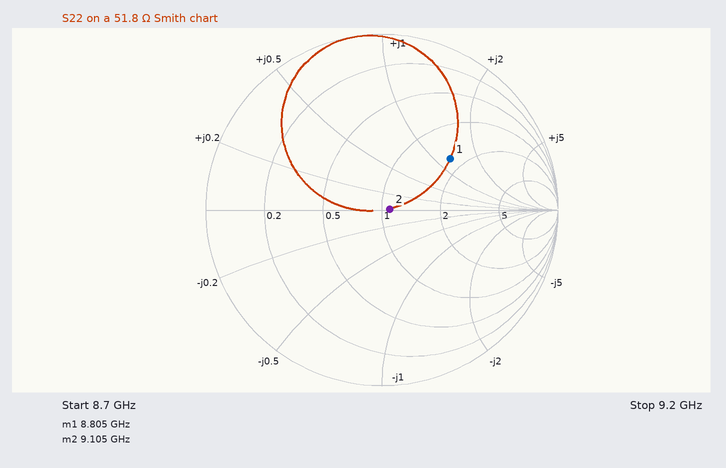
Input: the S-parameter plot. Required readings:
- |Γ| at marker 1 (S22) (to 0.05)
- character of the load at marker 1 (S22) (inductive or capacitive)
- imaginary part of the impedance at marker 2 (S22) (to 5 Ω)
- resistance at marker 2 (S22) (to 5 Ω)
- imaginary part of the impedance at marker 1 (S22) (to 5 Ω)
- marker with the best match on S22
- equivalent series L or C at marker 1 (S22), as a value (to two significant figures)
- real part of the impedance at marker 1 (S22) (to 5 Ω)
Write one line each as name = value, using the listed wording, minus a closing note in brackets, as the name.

|Γ| at marker 1 (S22) = 0.50
character of the load at marker 1 (S22) = inductive
imaginary part of the impedance at marker 2 (S22) = 0 Ω
resistance at marker 2 (S22) = 55 Ω
imaginary part of the impedance at marker 1 (S22) = +65 Ω
marker with the best match on S22 = marker 2
equivalent series L or C at marker 1 (S22), as a value = 1.2 nH
real part of the impedance at marker 1 (S22) = 85 Ω
